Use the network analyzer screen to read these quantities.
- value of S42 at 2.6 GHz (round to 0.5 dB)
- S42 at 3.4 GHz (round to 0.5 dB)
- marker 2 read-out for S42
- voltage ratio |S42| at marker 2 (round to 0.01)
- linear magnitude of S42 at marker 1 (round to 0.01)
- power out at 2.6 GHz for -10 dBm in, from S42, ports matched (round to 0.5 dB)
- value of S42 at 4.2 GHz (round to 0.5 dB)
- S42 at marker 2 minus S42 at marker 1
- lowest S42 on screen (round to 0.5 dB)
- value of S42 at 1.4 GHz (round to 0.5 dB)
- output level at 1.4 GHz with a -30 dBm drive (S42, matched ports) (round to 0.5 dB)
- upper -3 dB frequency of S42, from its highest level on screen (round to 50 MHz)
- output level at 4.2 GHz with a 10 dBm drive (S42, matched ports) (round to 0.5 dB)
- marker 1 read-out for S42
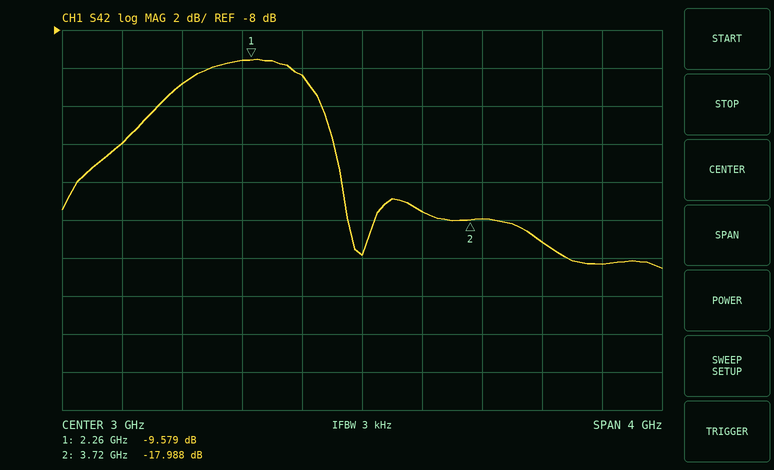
-10.5 dB
-17.5 dB
-17.988 dB
0.13
0.33
-20.5 dBm
-19.0 dB
-8.409 dB
-20.5 dB
-14.0 dB
-44.0 dBm
2.75 GHz
-9.0 dBm
-9.579 dB
